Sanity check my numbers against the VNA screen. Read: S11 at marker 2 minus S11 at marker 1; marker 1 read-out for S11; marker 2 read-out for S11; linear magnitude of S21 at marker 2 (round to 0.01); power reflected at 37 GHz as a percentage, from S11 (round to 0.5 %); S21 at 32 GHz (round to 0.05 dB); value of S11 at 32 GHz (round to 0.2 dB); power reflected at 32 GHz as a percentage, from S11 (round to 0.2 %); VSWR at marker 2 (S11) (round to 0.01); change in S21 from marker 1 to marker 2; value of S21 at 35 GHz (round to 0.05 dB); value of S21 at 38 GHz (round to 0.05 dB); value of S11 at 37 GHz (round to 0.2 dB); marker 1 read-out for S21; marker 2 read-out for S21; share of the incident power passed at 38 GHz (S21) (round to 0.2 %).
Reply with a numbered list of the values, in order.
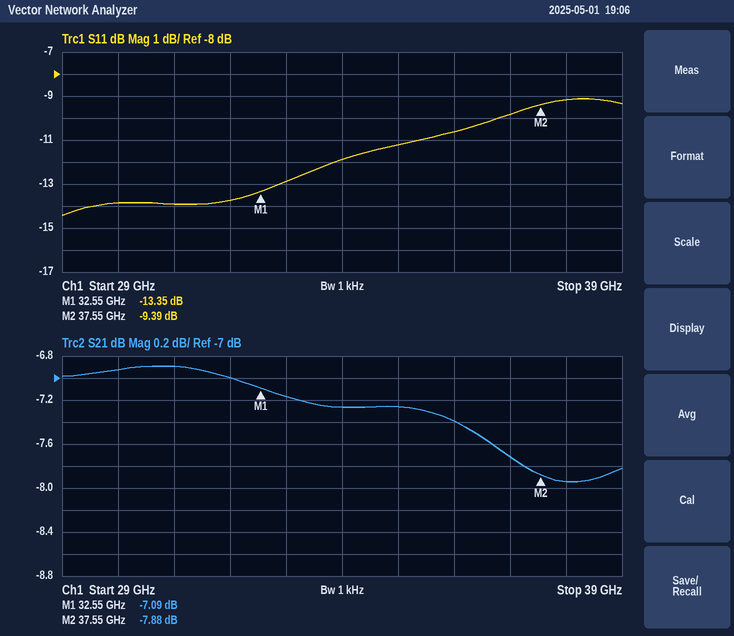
1. 3.96 dB
2. -13.35 dB
3. -9.39 dB
4. 0.40
5. 10.5 %
6. -7.00 dB
7. -13.8 dB
8. 4.2 %
9. 2.03
10. -0.79 dB
11. -7.25 dB
12. -7.95 dB
13. -9.8 dB
14. -7.09 dB
15. -7.88 dB
16. 16.0 %
